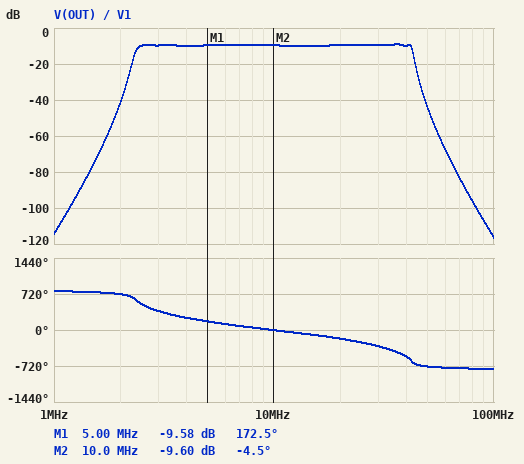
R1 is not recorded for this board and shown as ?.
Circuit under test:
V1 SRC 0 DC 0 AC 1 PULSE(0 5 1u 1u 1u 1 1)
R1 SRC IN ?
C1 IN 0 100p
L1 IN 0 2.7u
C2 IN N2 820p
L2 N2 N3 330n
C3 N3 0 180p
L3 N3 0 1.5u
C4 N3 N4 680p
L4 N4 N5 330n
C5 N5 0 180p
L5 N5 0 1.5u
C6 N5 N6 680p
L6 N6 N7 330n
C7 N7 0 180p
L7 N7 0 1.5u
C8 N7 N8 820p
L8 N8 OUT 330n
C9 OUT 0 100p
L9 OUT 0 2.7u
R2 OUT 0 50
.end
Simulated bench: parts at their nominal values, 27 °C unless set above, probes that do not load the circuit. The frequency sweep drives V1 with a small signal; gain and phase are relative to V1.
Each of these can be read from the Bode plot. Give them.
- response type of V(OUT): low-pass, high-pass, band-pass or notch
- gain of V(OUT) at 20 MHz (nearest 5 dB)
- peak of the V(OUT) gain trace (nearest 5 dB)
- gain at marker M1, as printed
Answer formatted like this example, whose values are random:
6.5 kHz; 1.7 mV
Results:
band-pass; -10 dB; -10 dB; -9.58 dB
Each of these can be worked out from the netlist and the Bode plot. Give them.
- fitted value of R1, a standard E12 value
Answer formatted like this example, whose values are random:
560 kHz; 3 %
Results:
100 Ω
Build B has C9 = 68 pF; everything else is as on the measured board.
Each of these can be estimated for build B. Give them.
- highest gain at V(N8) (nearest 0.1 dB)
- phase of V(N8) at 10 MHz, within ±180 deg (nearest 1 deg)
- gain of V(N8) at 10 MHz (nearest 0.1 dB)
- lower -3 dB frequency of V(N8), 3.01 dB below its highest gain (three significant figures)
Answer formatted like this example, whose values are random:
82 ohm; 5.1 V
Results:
-4.6 dB; 21 deg; -8.6 dB; 30.1 MHz
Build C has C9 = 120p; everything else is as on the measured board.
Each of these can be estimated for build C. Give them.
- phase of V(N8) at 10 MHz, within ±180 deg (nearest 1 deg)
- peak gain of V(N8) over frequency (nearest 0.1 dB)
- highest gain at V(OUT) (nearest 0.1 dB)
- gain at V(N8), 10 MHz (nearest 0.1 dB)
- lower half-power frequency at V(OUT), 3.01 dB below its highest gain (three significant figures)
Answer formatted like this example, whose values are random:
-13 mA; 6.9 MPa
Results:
16 deg; -2.2 dB; -9.1 dB; -9.2 dB; 2.37 MHz
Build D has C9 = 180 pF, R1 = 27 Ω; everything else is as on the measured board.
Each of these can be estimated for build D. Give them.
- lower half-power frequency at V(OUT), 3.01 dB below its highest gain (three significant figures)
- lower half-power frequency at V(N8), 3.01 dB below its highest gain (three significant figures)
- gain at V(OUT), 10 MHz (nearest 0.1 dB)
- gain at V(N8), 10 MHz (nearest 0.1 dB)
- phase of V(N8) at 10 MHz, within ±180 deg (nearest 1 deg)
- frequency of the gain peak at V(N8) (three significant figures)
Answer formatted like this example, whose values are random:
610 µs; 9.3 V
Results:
2.43 MHz; 40.3 MHz; -3.9 dB; -4.1 dB; 19 deg; 41.1 MHz
